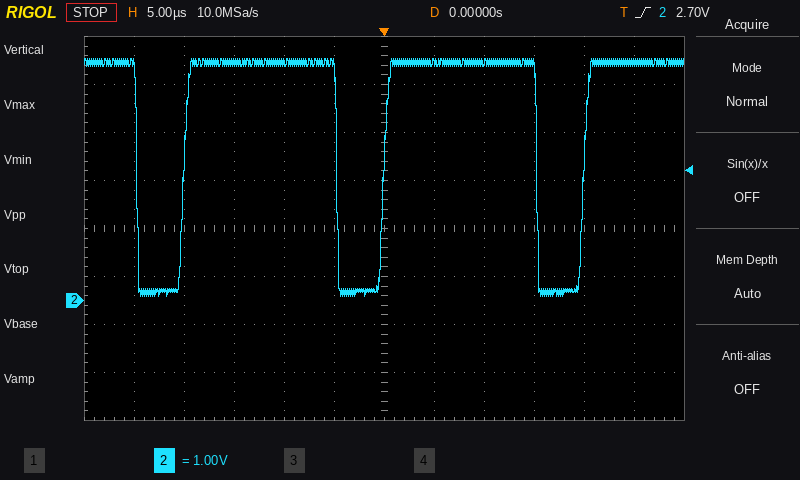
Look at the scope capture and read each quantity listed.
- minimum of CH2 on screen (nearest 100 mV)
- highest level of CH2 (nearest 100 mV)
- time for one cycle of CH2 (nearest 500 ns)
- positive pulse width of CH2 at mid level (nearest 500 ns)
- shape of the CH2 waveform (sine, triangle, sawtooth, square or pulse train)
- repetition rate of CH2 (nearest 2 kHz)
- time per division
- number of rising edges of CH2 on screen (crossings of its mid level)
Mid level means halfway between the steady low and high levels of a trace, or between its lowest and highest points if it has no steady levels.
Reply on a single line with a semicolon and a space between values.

100 mV; 5.0 V; 20.0 µs; 15.5 µs; pulse train; 50 kHz; 5 µs; 3
